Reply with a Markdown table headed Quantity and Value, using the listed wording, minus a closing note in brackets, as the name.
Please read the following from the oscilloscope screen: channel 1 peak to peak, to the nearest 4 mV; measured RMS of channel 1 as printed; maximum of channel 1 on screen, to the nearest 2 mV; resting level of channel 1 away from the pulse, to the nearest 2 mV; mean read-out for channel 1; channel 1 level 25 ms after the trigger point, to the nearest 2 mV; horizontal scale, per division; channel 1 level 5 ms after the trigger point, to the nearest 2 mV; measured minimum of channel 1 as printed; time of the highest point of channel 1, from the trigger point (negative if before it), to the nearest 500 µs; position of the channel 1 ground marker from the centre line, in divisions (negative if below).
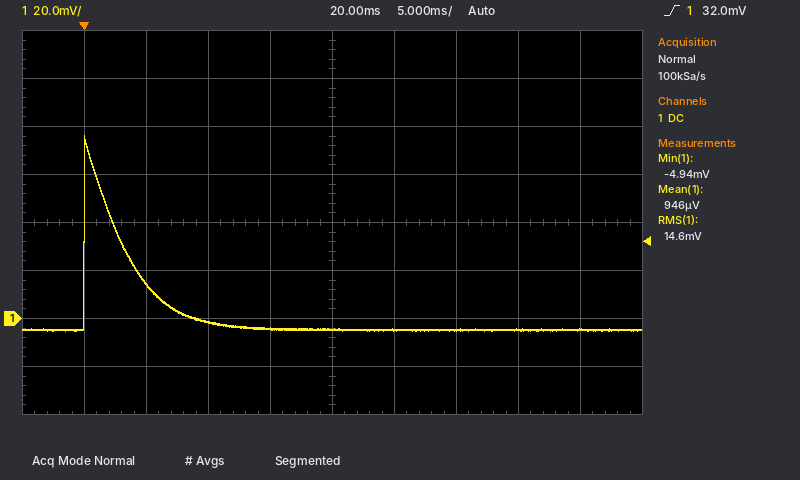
| Quantity | Value |
|---|---|
| channel 1 peak to peak, to the nearest 4 mV | 80 mV |
| measured RMS of channel 1 as printed | 14.6 mV |
| maximum of channel 1 on screen, to the nearest 2 mV | 76 mV |
| resting level of channel 1 away from the pulse, to the nearest 2 mV | -4 mV |
| mean read-out for channel 1 | 946 µV |
| channel 1 level 25 ms after the trigger point, to the nearest 2 mV | -4 mV |
| horizontal scale, per division | 5 ms |
| channel 1 level 5 ms after the trigger point, to the nearest 2 mV | 14 mV |
| measured minimum of channel 1 as printed | -4.94 mV |
| time of the highest point of channel 1, from the trigger point (negative if before it), to the nearest 500 µs | 0.0 ms |
| position of the channel 1 ground marker from the centre line, in divisions | -2.0 div |
